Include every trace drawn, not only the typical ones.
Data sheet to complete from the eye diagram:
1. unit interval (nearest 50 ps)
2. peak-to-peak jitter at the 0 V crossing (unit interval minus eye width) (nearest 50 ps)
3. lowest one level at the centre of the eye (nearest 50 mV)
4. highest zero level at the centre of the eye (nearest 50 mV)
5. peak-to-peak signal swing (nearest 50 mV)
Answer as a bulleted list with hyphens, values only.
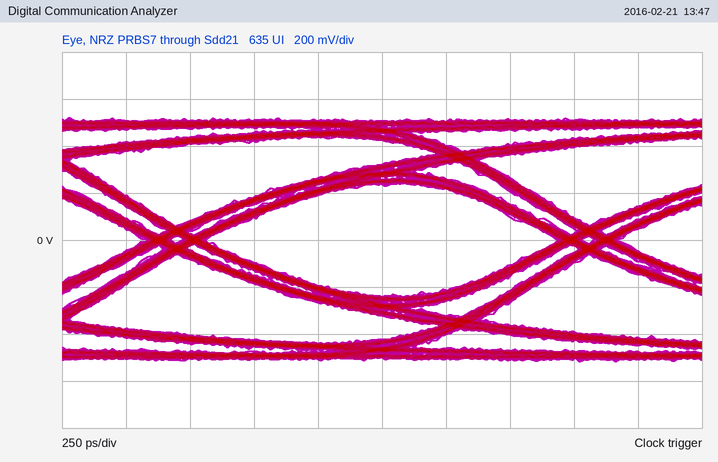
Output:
- 1.60 ns
- 250 ps
- 250 mV
- -250 mV
- 1.05 V
